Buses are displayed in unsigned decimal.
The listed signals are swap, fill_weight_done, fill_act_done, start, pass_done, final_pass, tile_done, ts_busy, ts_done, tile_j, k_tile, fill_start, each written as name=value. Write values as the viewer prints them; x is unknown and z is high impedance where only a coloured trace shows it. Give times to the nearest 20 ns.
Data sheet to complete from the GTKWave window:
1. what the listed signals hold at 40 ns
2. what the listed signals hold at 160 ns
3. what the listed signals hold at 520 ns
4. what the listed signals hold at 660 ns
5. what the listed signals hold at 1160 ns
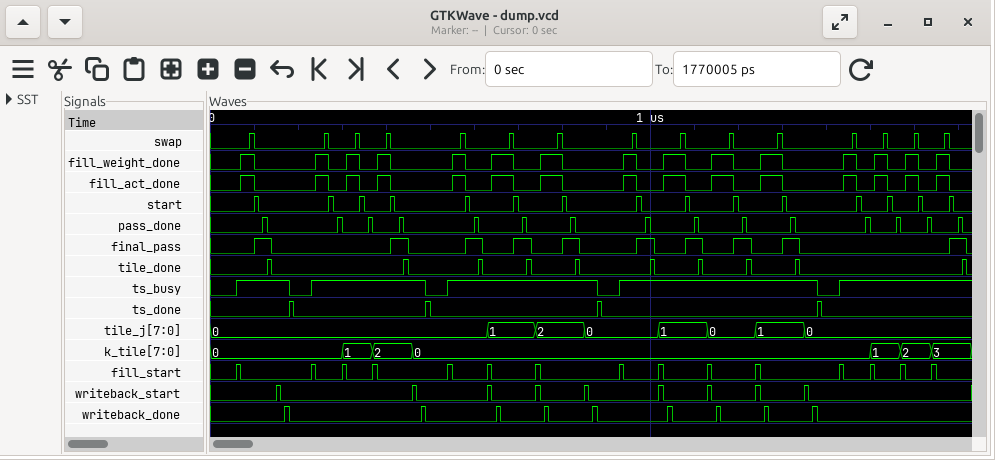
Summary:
swap=0, fill_weight_done=0, fill_act_done=0, start=0, pass_done=0, final_pass=0, tile_done=0, ts_busy=0, ts_done=0, tile_j=0, k_tile=0, fill_start=0
swap=0, fill_weight_done=0, fill_act_done=0, start=0, pass_done=0, final_pass=0, tile_done=0, ts_busy=1, ts_done=0, tile_j=0, k_tile=0, fill_start=0
swap=0, fill_weight_done=0, fill_act_done=0, start=0, pass_done=0, final_pass=0, tile_done=0, ts_busy=0, ts_done=0, tile_j=0, k_tile=0, fill_start=0
swap=0, fill_weight_done=1, fill_act_done=1, start=0, pass_done=0, final_pass=0, tile_done=0, ts_busy=1, ts_done=0, tile_j=1, k_tile=0, fill_start=0
swap=0, fill_weight_done=1, fill_act_done=1, start=0, pass_done=0, final_pass=0, tile_done=0, ts_busy=1, ts_done=0, tile_j=0, k_tile=0, fill_start=0
